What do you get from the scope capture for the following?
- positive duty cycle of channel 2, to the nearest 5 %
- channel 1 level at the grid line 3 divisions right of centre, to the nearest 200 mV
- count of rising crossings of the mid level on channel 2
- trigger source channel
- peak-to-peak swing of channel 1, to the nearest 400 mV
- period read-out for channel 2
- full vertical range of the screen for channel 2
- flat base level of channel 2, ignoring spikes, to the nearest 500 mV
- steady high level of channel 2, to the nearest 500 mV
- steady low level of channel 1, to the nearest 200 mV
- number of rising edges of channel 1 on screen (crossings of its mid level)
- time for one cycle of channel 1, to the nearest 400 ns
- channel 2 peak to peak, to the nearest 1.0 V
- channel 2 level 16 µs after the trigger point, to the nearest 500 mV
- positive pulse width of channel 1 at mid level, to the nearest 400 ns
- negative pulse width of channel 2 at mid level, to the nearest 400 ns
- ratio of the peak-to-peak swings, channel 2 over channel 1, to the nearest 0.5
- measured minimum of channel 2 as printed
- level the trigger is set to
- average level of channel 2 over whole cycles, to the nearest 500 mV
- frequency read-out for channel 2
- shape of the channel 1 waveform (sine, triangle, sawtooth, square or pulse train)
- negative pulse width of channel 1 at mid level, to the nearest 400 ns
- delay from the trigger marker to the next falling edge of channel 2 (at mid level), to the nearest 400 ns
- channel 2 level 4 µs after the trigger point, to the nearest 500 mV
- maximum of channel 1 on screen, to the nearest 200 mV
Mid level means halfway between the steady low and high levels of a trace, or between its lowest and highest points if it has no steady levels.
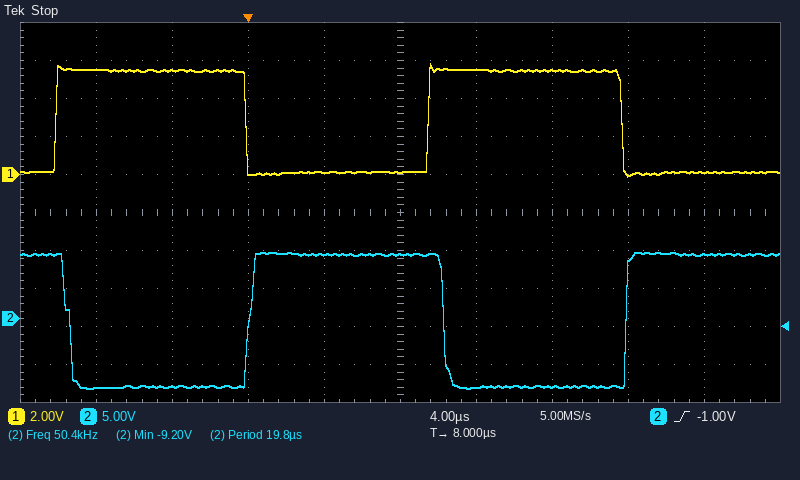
50 %
0.0 V
2
channel 2
6.0 V
19.8 µs
50 V
-9.0 V
8.5 V
200 mV
2
19.6 µs
18.0 V
-9.0 V
10.0 µs
9.6 µs
3.0
-9.20 V
-1.00 V
0.0 V
50.4 kHz
square
9.6 µs
10.4 µs
8.5 V
5.8 V
